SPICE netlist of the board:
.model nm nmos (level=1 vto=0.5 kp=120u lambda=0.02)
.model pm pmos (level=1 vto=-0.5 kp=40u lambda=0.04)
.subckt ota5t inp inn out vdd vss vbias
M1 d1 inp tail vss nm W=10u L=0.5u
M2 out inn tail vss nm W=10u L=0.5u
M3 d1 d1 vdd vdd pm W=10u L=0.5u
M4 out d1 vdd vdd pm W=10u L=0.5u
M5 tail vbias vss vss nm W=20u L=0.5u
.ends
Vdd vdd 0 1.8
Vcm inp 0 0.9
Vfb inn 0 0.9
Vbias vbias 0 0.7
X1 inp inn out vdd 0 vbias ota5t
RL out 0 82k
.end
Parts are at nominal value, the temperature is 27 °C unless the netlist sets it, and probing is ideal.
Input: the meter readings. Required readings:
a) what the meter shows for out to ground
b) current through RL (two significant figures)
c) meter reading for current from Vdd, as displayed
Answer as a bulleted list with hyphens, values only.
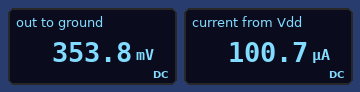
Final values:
- 353.8 mV
- 4.3 µA
- 100.7 µA
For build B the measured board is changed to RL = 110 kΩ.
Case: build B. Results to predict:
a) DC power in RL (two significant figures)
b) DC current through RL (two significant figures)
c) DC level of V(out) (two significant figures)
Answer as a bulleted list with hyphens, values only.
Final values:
- 1.2 µW
- 3.3 µA
- 360 mV
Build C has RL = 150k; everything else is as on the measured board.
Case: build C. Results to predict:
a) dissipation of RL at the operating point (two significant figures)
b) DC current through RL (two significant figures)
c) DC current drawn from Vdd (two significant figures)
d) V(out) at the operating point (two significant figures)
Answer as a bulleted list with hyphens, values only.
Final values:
- 930 nW
- 2.5 µA
- 99 µA
- 370 mV
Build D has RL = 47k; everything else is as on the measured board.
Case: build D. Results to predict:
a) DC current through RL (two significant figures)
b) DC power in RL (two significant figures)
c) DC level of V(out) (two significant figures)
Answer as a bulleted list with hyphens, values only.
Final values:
- 7.1 µA
- 2.4 µW
- 330 mV
